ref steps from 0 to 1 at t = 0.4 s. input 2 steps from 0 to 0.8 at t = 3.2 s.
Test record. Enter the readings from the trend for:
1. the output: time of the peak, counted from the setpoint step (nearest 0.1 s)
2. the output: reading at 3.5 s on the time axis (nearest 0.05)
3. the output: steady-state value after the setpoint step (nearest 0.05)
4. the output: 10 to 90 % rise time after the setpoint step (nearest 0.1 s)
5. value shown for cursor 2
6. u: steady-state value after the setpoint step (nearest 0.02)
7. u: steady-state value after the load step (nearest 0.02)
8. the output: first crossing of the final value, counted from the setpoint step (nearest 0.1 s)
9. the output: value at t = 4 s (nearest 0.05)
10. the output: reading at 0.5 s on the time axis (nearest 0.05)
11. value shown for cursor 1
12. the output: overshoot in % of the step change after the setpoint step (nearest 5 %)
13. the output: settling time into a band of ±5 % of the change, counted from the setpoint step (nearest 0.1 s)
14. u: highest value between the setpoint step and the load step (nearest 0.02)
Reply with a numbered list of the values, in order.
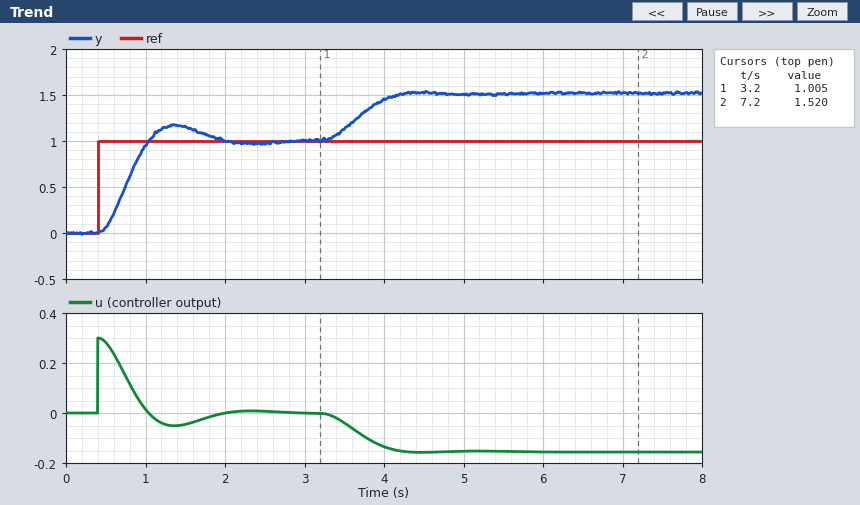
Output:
1. 1.0 s
2. 1.15
3. 1.00
4. 0.4 s
5. 1.520
6. 0.00
7. -0.16
8. 0.6 s
9. 1.45
10. 0.05
11. 1.005
12. 15 %
13. 1.4 s
14. 0.30
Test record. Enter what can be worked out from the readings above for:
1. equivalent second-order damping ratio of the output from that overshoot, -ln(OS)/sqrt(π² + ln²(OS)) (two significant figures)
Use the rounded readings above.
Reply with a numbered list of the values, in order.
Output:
1. 0.52
